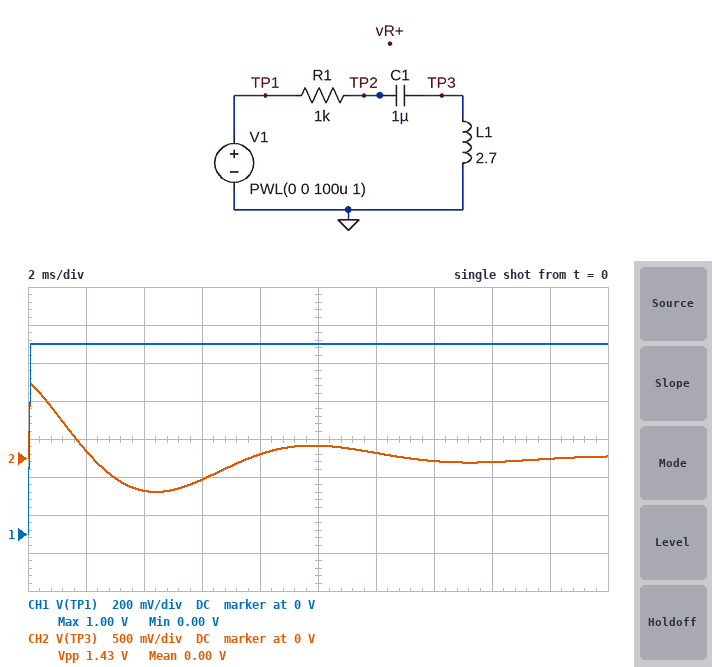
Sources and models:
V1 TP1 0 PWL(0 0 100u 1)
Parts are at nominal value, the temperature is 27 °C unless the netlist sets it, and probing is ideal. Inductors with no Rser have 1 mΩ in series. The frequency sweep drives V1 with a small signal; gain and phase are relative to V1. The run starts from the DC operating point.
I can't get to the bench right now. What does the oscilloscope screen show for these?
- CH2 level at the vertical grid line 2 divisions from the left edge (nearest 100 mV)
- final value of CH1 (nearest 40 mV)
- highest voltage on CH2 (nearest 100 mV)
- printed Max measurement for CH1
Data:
-400 mV
1.00 V
1.0 V
1.00 V
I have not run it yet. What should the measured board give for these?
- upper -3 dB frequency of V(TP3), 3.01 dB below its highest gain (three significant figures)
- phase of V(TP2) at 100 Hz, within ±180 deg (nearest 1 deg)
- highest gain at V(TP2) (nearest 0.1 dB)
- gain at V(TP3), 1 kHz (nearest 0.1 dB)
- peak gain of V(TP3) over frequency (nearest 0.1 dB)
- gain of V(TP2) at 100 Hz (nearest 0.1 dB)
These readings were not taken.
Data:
200 Hz
84 deg
0 dB
0.1 dB
4.7 dB
-19.6 dB
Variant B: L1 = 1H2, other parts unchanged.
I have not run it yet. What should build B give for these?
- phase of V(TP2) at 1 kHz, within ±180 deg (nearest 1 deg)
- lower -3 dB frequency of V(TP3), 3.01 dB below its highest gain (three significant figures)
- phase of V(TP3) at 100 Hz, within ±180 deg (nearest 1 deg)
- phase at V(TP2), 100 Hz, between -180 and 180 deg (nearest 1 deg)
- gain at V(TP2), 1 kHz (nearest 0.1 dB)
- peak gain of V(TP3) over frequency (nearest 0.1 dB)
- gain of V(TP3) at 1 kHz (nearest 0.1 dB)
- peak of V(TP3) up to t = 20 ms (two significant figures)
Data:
8 deg
123 Hz
130 deg
-50 deg
-0.1 dB
1.8 dB
0.1 dB
960 mV
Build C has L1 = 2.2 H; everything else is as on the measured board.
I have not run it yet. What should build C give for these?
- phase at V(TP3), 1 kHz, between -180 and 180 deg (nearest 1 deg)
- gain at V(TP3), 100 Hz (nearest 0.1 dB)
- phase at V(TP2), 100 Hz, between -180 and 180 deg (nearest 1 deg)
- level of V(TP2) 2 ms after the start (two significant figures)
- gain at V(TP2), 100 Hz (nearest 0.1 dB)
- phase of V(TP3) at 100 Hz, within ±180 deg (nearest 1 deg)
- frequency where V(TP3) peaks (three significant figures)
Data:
4 deg
2.6 dB
-78 deg
570 mV
-13.8 dB
102 deg
122 Hz
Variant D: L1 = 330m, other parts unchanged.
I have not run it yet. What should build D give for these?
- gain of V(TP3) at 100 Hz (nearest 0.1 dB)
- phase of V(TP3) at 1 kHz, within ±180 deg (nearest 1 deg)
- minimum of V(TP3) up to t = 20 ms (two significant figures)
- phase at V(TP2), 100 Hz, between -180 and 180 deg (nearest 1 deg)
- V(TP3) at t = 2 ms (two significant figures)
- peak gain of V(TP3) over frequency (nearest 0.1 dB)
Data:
-18.3 dB
28 deg
-160 mV
-36 deg
-97 mV
0 dB
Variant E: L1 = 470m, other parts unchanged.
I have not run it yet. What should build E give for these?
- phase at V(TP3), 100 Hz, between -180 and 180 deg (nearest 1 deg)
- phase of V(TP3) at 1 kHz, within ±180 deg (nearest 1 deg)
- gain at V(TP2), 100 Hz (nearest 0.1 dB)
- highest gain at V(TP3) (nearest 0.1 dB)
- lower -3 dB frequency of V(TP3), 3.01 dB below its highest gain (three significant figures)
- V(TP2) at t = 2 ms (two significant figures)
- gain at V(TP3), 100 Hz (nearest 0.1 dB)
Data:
142 deg
20 deg
-2.0 dB
0 dB
240 Hz
750 mV
-14.9 dB
